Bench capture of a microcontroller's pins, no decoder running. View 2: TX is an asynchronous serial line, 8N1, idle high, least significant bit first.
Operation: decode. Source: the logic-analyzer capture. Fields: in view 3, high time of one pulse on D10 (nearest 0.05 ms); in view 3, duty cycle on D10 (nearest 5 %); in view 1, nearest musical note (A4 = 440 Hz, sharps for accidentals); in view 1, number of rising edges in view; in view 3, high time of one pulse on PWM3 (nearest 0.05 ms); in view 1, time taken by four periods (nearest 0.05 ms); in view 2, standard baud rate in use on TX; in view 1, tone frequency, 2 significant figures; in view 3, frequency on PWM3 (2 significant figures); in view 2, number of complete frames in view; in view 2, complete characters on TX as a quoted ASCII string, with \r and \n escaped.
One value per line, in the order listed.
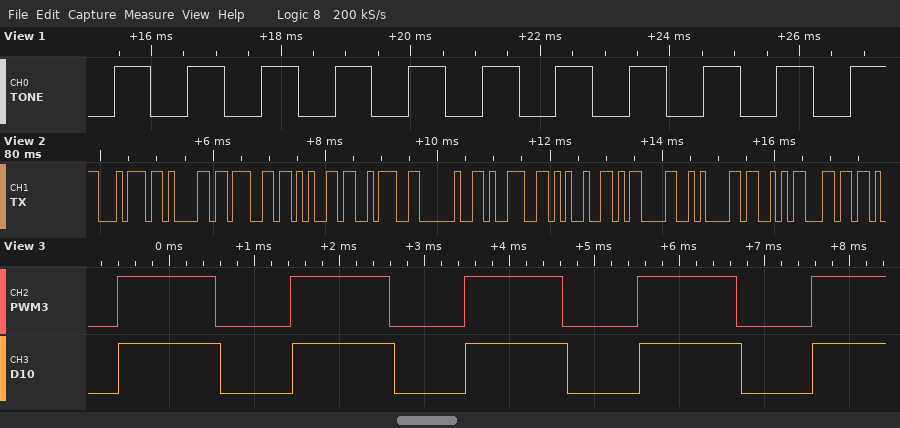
1.20 ms
60 %
A5
11
1.15 ms
4.55 ms
9600 baud
880 Hz
490 Hz
12
"tage: 9%\r\nSl"
